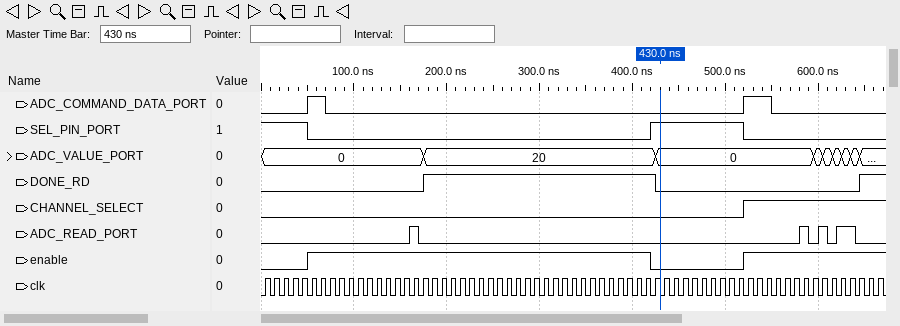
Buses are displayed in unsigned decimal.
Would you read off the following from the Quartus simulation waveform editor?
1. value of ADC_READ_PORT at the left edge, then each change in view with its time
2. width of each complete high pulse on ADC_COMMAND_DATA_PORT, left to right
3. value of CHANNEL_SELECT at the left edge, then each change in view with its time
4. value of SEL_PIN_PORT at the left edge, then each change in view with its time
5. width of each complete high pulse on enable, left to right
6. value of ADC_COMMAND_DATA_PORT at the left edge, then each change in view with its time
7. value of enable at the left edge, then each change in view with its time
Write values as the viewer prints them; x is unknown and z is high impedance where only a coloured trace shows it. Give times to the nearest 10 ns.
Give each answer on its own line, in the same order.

0, 1 at 160 ns, 0 at 170 ns, 1 at 580 ns, 0 at 590 ns, 1 at 600 ns, 0 at 610 ns, 1 at 620 ns, 0 at 640 ns
20 ns, 30 ns
0, 1 at 520 ns
1, 0 at 50 ns, 1 at 420 ns, 0 at 520 ns
370 ns
0, 1 at 50 ns, 0 at 70 ns, 1 at 520 ns, 0 at 550 ns
0, 1 at 50 ns, 0 at 420 ns, 1 at 520 ns
